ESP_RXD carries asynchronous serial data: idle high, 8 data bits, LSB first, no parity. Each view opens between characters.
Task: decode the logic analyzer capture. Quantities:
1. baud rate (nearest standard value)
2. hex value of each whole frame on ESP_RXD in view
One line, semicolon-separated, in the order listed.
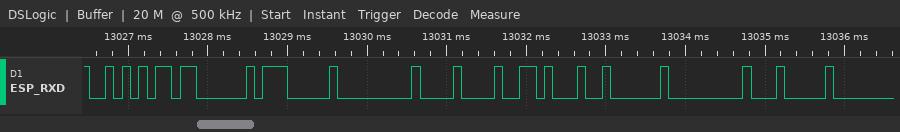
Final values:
9600 baud; AA, 03, 07, 00, 08, 16, 02, 00, 04
